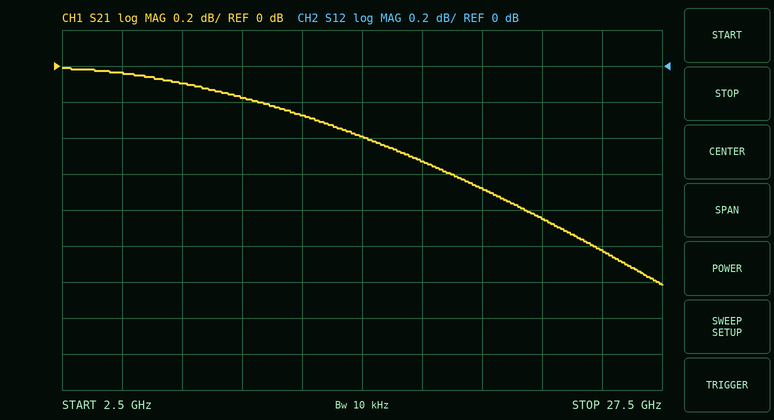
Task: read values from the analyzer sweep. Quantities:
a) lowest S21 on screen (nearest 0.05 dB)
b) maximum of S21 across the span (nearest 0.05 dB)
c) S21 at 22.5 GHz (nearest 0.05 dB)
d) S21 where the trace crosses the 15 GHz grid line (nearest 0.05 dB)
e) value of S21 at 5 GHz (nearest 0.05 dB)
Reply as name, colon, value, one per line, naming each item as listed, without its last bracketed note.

lowest S21 on screen: -1.20 dB
maximum of S21 across the span: 0.00 dB
S21 at 22.5 GHz: -0.85 dB
S21 where the trace crosses the 15 GHz grid line: -0.40 dB
value of S21 at 5 GHz: -0.05 dB
